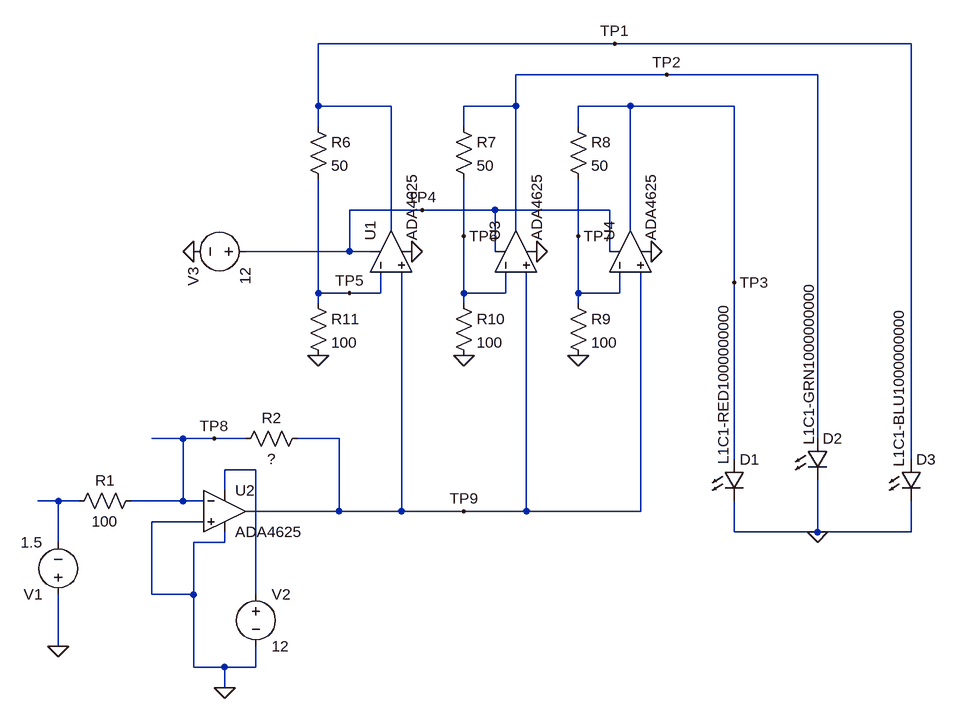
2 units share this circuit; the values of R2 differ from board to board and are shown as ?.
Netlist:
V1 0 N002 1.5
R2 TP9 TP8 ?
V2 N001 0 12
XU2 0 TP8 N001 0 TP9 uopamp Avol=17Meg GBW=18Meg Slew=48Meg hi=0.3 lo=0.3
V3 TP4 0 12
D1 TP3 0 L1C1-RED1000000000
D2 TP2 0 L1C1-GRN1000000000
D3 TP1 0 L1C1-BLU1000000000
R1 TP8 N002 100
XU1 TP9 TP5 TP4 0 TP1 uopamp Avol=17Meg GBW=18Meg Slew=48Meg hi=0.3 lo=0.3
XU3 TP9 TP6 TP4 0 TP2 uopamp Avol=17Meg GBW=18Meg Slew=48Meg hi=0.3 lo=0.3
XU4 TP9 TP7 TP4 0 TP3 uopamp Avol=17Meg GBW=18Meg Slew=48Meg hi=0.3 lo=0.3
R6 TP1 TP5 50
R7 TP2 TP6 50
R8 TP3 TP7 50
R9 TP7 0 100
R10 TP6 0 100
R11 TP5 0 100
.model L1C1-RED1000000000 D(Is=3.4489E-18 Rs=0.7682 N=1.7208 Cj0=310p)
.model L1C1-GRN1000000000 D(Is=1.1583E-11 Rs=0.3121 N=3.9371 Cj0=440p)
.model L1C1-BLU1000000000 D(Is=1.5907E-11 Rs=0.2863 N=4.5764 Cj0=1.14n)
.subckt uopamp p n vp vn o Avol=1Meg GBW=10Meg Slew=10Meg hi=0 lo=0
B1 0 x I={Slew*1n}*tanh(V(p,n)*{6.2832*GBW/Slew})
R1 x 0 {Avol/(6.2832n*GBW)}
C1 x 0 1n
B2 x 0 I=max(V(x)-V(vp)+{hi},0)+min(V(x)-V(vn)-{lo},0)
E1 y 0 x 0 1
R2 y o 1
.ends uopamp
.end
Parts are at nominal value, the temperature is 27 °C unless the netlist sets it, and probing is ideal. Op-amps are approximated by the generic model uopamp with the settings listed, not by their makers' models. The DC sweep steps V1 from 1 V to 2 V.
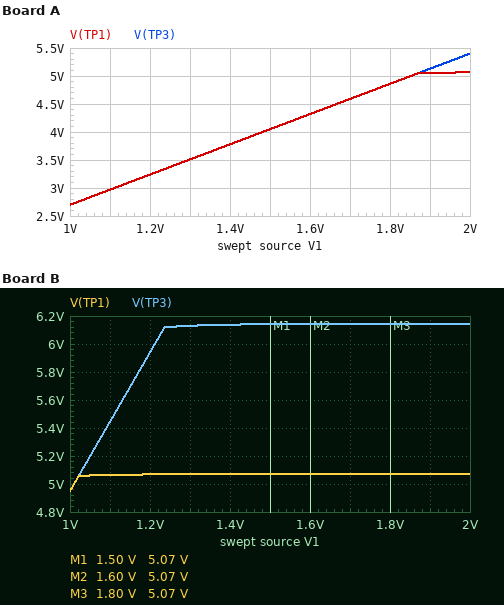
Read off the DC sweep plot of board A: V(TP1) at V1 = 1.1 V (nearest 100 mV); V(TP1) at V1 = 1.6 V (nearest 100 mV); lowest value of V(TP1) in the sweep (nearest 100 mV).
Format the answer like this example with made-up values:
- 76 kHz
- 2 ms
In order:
- 3.0 V
- 4.3 V
- 2.7 V
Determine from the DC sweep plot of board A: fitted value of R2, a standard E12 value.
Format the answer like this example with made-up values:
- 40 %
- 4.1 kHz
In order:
- 180 Ω
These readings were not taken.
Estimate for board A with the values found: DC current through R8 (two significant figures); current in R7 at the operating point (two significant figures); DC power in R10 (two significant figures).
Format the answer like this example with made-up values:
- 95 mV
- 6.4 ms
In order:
- 27 mA
- 27 mA
- 73 mW
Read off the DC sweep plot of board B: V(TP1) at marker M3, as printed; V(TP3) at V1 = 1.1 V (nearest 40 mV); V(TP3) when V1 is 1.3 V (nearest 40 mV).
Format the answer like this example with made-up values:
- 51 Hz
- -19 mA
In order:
- 5.07 V
- 5.44 V
- 6.12 V
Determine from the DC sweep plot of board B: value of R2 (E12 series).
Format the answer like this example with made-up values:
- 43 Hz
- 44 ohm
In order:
- 330 Ω
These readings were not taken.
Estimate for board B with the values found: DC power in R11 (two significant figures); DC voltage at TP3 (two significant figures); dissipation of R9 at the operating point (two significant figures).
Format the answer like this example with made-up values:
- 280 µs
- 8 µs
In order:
- 110 mW
- 6.1 V
- 170 mW
